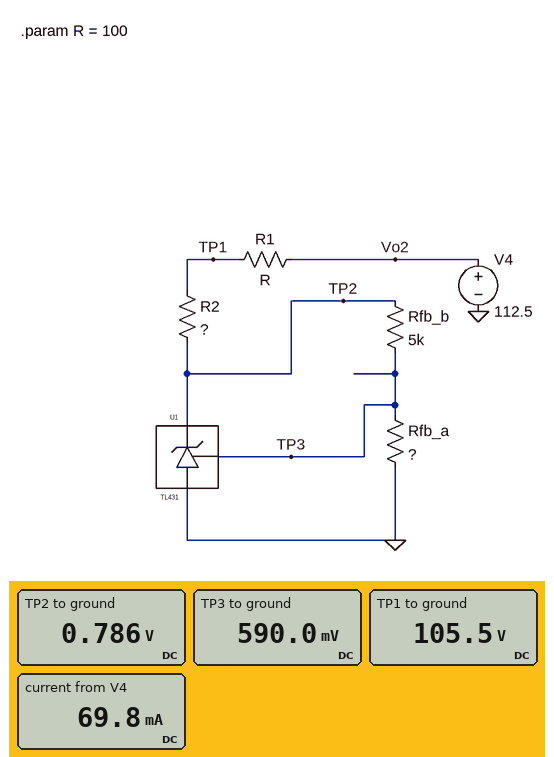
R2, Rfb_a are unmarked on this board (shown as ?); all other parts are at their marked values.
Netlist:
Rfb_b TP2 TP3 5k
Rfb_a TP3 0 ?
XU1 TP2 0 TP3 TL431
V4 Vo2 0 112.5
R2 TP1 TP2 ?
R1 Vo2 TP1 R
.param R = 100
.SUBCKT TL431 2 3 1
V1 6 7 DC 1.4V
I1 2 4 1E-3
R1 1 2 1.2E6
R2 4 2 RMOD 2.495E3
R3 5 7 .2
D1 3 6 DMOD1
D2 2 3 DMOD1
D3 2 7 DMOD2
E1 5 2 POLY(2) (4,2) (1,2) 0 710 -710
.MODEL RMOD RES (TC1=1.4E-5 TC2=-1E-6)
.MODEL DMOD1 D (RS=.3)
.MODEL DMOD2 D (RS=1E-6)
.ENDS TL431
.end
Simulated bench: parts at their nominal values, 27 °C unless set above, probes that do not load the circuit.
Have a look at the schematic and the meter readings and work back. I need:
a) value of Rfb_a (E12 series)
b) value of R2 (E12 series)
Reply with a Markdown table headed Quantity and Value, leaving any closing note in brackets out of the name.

| Quantity | Value |
|---|---|
| value of Rfb_a | 15 kΩ |
| value of R2 | 1.5 kΩ |
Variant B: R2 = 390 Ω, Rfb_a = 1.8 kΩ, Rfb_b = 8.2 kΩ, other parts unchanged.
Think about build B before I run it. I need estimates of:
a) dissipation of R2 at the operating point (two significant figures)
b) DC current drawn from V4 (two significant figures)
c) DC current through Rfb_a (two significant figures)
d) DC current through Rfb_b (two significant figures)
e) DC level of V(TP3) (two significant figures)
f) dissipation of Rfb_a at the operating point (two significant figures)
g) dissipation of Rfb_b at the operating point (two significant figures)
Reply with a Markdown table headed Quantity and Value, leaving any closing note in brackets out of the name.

| Quantity | Value |
|---|---|
| dissipation of R2 at the operating point | 20 W |
| DC current drawn from V4 | 230 mA |
| DC current through Rfb_a | 87 µA |
| DC current through Rfb_b | 86 µA |
| DC level of V(TP3) | 160 mV |
| dissipation of Rfb_a at the operating point | 14 µW |
| dissipation of Rfb_b at the operating point | 61 µW |
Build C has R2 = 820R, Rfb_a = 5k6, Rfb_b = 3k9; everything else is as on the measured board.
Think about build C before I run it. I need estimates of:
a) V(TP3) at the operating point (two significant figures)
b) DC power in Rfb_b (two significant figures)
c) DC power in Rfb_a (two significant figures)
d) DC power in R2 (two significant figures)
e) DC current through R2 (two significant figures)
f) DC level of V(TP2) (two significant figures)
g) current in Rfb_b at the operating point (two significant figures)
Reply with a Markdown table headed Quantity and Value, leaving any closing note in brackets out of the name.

| Quantity | Value |
|---|---|
| V(TP3) at the operating point | 480 mV |
| DC power in Rfb_b | 29 µW |
| DC power in Rfb_a | 41 µW |
| DC power in R2 | 12 W |
| DC current through R2 | 120 mA |
| DC level of V(TP2) | 820 mV |
| current in Rfb_b at the operating point | 86 µA |
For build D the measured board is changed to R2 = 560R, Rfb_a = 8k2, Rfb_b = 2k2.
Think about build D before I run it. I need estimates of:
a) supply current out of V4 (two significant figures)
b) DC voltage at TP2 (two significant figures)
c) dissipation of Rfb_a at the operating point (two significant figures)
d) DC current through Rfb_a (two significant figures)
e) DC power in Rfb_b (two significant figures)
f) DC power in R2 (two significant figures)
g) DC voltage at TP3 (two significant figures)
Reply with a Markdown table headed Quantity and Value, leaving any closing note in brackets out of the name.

| Quantity | Value |
|---|---|
| supply current out of V4 | 170 mA |
| DC voltage at TP2 | 840 mV |
| dissipation of Rfb_a at the operating point | 53 µW |
| DC current through Rfb_a | 81 µA |
| DC power in Rfb_b | 14 µW |
| DC power in R2 | 16 W |
| DC voltage at TP3 | 660 mV |
